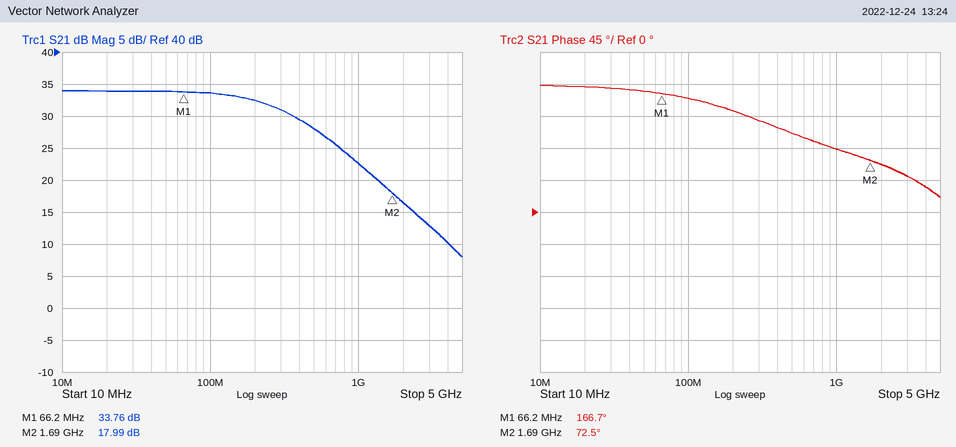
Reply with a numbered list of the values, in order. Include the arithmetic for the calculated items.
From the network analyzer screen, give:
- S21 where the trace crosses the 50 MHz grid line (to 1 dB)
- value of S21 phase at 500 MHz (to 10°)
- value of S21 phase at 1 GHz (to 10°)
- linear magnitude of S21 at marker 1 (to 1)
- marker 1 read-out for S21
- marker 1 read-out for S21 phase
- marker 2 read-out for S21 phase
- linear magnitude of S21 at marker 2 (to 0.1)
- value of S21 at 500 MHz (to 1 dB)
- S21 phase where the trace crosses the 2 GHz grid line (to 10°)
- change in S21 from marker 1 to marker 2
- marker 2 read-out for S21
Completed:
1. 34 dB
2. 110°
3. 90°
4. 10^(33.76/20) ≈ 49
5. 33.76 dB
6. 166.7°
7. 72.5°
8. 10^(17.99/20) ≈ 7.9
9. 28 dB
10. 70°
11. 17.99 − (33.76) = -15.77 dB
12. 17.99 dB
